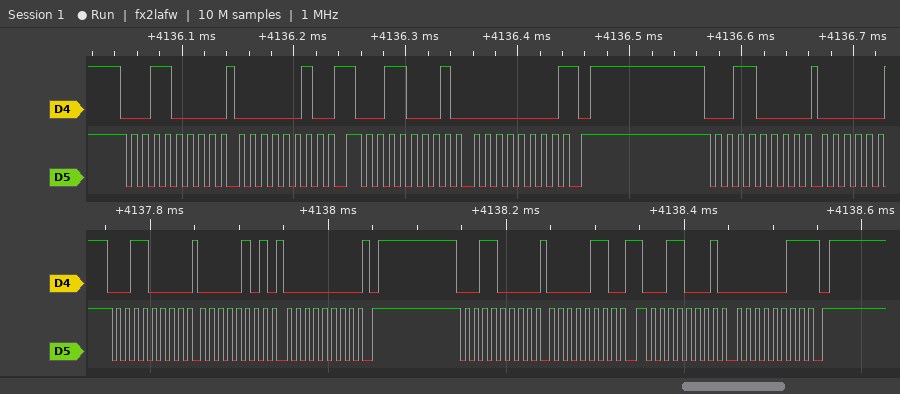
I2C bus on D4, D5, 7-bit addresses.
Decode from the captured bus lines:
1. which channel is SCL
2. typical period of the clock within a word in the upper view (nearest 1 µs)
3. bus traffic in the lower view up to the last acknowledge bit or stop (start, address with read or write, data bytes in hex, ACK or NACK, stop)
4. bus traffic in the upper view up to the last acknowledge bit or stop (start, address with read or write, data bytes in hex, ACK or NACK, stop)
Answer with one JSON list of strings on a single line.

["D5", "10 µs", "start, address 18 write ACK, 05 ACK, 00 ACK, stop, start, address 18 write ACK, 06 ACK, repeated start, address 18 read ACK, 03 NACK, stop", "start, address 18 write ACK, 02 ACK, repeated start, address 18 read ACK, 00 NACK, stop, start, address 18 write ACK"]
